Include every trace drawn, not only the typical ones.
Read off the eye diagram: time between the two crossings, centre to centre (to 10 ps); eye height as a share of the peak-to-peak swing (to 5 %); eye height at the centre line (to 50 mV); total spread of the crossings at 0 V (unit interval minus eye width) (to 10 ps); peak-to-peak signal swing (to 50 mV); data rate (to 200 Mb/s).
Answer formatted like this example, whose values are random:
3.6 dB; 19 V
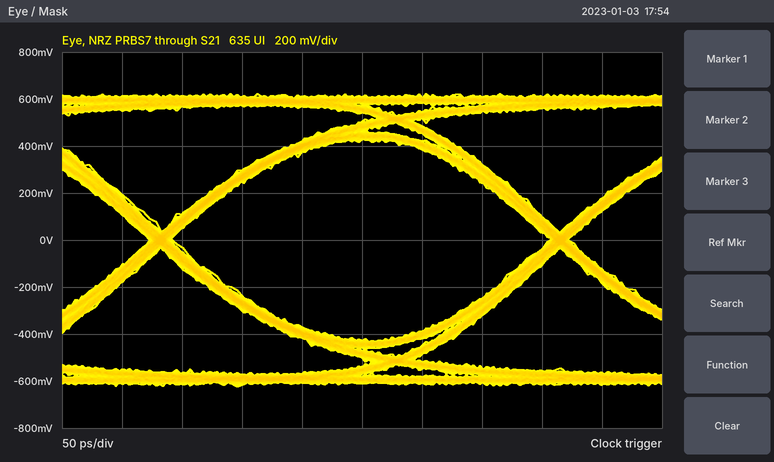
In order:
330 ps; 70 %; 850 mV; 20 ps; 1.25 V; 3.0 Gb/s
